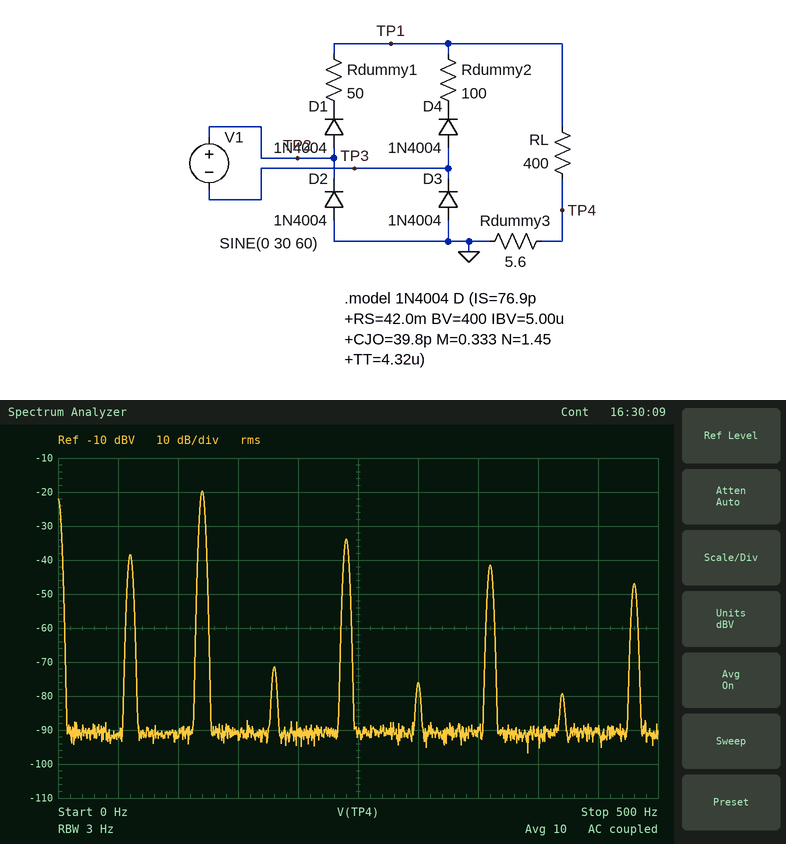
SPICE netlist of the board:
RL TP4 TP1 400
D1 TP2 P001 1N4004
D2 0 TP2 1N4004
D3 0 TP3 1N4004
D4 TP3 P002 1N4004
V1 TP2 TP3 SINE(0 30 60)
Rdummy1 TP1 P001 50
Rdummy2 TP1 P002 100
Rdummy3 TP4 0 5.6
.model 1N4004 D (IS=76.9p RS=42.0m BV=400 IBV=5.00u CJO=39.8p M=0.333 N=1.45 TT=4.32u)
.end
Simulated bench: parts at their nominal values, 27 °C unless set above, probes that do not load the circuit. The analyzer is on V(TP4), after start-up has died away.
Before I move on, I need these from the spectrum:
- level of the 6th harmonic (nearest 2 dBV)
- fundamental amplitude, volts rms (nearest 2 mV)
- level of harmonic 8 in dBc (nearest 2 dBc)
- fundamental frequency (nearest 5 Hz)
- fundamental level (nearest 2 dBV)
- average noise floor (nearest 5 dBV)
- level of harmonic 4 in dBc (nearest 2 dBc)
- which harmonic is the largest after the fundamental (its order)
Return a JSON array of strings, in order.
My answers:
["-42 dBV", "12 mV", "-8 dBc", "60 Hz", "-38 dBV", "-90 dBV", "4 dBc", "2"]
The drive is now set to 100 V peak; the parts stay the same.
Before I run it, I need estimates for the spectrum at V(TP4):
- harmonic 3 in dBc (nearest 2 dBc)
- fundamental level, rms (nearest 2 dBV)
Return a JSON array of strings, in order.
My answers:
["-44 dBc", "-28 dBV"]
